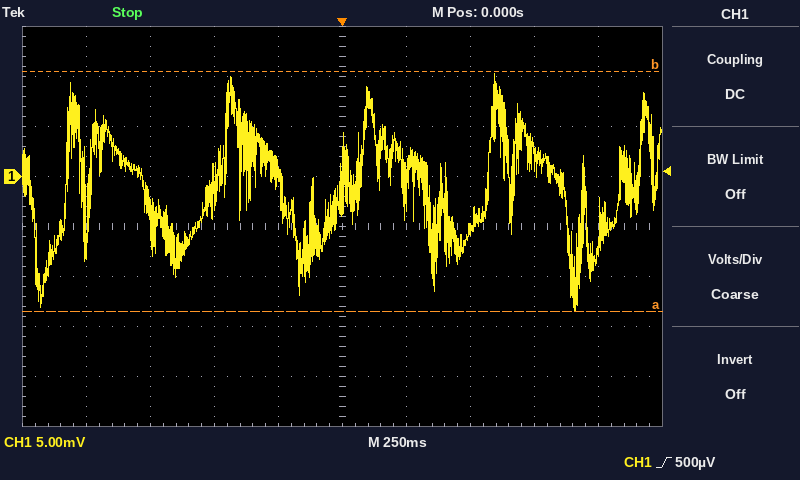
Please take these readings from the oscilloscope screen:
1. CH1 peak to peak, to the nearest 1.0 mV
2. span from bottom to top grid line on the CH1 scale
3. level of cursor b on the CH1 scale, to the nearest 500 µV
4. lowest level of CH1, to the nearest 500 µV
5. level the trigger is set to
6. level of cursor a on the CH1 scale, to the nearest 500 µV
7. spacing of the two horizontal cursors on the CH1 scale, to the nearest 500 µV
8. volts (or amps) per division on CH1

24.0 mV
40 mV
10.5 mV
-13.5 mV
500 µV
-13.5 mV
24.0 mV
5 mV
